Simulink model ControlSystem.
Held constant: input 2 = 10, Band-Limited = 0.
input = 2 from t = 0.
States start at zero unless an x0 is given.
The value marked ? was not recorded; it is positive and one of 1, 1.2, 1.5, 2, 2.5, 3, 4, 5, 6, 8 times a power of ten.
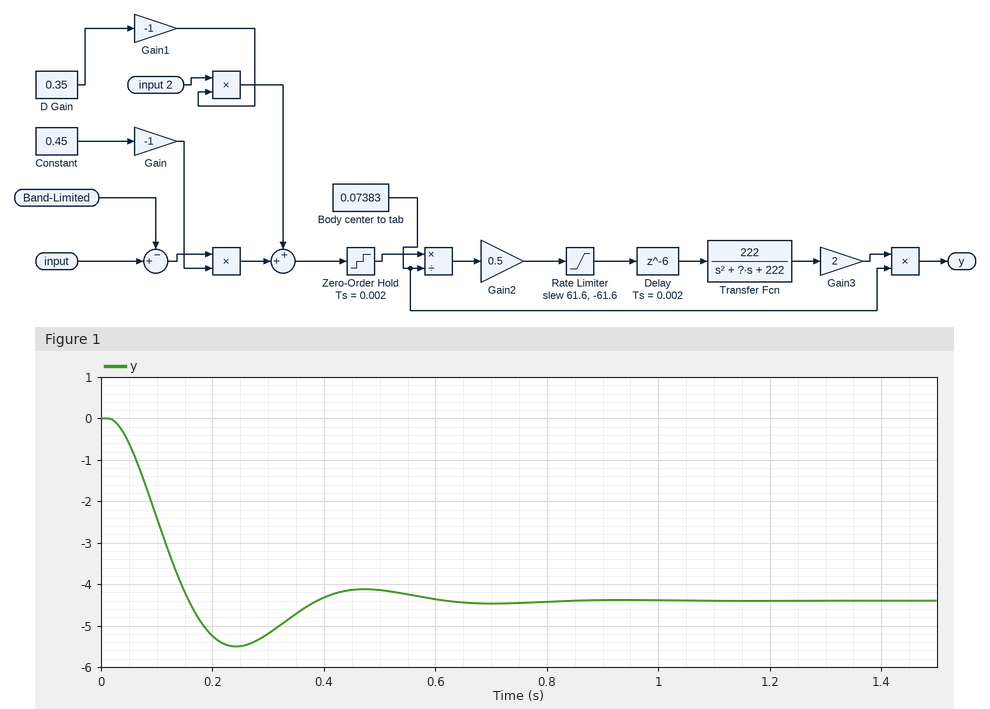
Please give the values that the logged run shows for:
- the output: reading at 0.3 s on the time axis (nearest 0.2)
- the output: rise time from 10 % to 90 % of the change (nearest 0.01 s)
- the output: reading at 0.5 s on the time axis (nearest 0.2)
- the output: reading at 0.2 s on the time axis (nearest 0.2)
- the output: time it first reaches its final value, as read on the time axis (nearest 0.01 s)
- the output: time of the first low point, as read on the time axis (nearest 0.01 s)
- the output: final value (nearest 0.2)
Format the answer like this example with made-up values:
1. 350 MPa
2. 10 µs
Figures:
1. -5.2
2. 0.10 s
3. -4.2
4. -5.2
5. 0.16 s
6. 0.24 s
7. -4.4
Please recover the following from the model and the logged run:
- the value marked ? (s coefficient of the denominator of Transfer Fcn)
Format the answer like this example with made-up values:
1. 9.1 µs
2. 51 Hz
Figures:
1. 12
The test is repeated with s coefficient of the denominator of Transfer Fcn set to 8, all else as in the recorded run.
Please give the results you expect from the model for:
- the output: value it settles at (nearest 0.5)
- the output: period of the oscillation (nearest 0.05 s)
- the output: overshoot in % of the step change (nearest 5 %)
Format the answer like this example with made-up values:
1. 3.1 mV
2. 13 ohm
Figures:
1. -4.5
2. 0.45 s
3. 40 %
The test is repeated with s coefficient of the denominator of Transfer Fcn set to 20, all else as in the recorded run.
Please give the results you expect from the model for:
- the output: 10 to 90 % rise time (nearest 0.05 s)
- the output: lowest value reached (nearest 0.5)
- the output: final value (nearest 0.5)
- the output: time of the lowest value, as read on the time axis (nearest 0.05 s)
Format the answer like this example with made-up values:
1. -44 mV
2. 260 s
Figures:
1. 0.15 s
2. -4.5
3. -4.5
4. 0.30 s
